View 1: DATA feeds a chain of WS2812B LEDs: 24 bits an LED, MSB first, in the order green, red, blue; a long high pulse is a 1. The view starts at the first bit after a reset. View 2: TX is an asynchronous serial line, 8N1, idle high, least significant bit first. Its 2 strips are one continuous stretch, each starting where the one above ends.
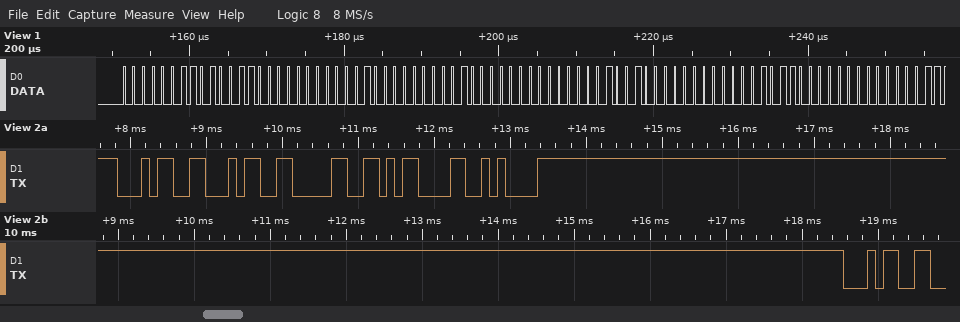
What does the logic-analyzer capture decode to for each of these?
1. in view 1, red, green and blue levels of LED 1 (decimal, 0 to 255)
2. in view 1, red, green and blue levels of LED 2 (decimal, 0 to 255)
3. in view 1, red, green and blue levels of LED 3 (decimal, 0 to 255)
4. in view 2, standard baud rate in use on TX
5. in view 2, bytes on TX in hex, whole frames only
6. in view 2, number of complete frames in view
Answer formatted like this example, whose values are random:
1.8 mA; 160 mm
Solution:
76, 3, 0; 16, 64, 0; 0, 36, 44; 9600 baud; 34 34 30 0D 0A 34; 6
